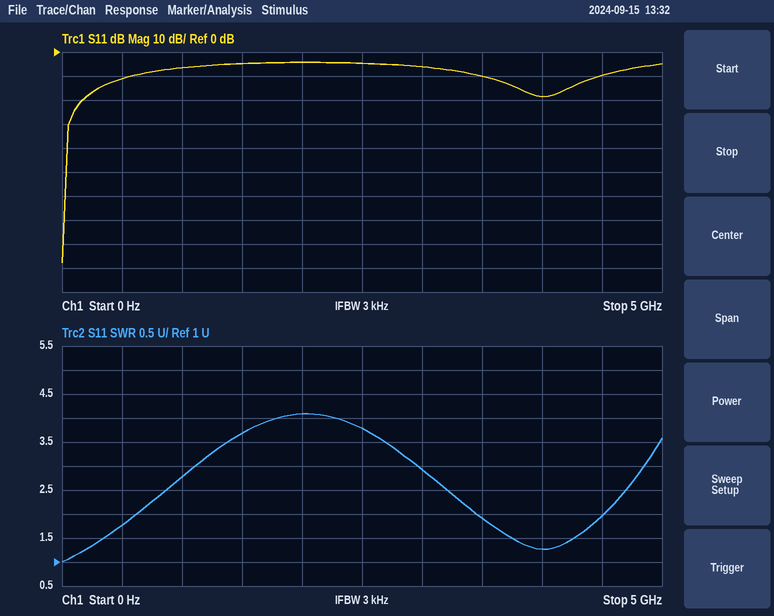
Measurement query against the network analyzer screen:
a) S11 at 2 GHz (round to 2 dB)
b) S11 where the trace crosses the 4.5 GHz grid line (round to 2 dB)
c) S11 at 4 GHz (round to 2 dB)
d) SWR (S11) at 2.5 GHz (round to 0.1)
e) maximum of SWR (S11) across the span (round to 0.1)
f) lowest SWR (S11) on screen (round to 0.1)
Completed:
-4 dB
-10 dB
-18 dB
3.8
4.1
1.0
